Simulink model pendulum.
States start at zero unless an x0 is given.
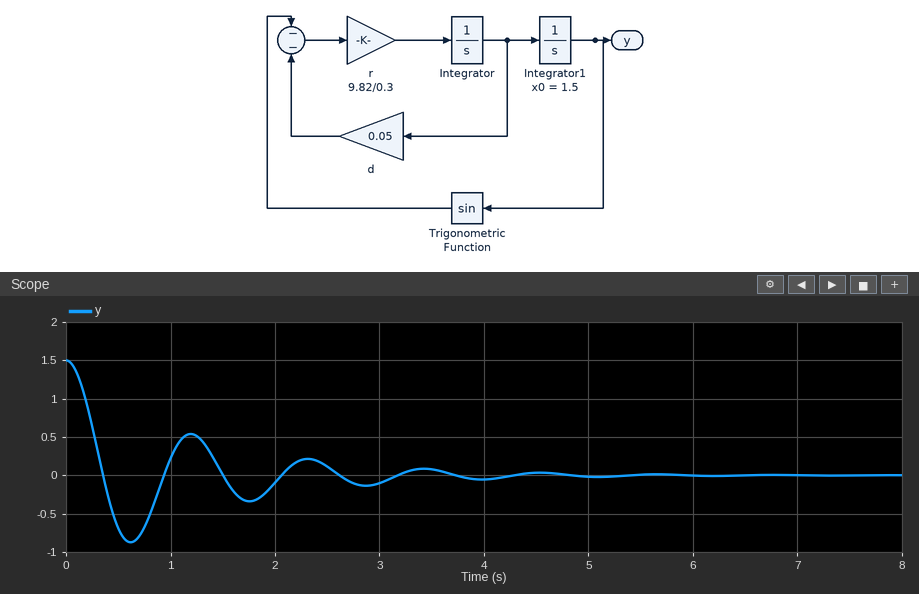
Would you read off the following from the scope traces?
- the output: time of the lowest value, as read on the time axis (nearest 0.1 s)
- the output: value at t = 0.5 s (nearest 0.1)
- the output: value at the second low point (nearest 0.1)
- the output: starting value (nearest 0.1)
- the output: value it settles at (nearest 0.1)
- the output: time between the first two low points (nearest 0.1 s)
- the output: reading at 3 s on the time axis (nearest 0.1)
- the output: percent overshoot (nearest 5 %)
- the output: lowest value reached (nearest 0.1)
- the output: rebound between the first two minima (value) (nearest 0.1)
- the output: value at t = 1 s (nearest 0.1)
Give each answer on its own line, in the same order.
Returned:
0.6 s
-0.7
-0.3
1.5
0.0
1.1 s
-0.1
60 %
-0.9
0.5
0.2
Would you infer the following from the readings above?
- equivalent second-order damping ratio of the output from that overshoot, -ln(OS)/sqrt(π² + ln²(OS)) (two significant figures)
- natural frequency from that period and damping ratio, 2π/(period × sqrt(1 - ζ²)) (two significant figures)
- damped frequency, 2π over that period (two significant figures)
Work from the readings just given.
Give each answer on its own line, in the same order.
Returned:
0.16
5.8 rad/s
5.7 rad/s
